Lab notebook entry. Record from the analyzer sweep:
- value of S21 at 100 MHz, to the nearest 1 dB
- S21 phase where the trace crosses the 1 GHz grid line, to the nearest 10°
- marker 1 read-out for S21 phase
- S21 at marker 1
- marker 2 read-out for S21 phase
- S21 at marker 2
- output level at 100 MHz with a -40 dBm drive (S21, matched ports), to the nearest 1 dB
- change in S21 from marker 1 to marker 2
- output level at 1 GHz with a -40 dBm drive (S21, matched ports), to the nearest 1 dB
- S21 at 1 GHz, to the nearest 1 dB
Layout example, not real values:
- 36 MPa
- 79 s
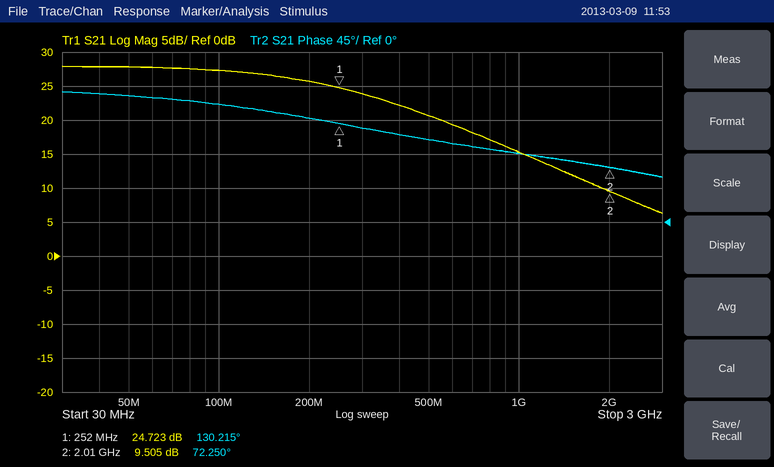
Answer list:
- 27 dB
- 90°
- 130.215°
- 24.723 dB
- 72.250°
- 9.505 dB
- -13 dBm
- -15.218 dB
- -25 dBm
- 15 dB
